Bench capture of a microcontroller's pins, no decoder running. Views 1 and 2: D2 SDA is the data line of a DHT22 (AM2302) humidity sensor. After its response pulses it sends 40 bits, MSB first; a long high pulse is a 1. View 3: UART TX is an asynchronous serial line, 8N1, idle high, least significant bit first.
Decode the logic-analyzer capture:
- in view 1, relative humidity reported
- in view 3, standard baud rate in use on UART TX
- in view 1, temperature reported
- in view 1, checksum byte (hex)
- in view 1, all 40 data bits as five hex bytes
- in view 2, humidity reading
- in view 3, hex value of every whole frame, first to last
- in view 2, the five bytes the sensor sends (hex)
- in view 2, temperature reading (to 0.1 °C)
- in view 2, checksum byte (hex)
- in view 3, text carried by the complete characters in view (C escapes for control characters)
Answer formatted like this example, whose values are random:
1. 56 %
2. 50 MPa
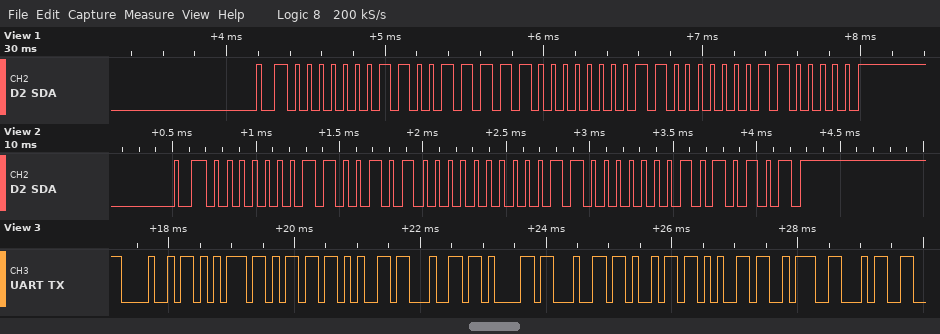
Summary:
1. 41.5 %
2. 9600 baud
3. 19.2 °C
4. 0x60
5. 01 9F 00 C0 60
6. 40.4 %
7. 48 75 6D 65 64 61 64 69 65 3A 34
8. 01 94 00 C0 55
9. 19.2 °C
10. 0x55
11. "Humedadie:4"
